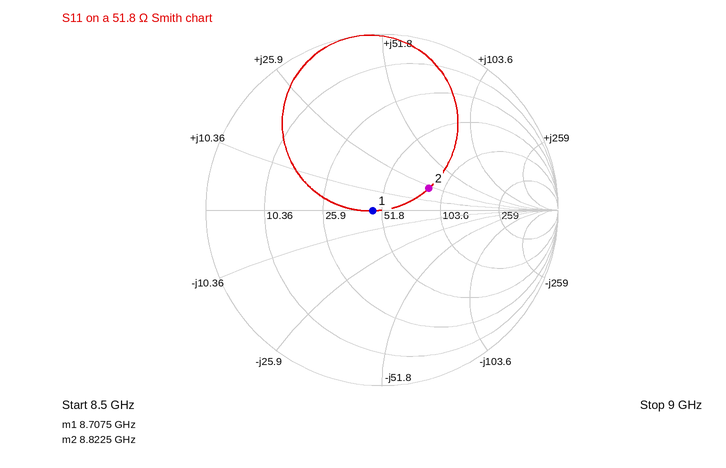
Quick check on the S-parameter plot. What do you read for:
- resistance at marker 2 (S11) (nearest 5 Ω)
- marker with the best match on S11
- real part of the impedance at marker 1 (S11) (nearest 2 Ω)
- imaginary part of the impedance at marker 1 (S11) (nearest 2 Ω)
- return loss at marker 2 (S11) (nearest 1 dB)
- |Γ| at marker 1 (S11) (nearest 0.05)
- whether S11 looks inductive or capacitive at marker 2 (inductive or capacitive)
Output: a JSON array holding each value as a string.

["85 Ω", "marker 1", "46 Ω", "0 Ω", "11 dB", "0.05", "inductive"]
